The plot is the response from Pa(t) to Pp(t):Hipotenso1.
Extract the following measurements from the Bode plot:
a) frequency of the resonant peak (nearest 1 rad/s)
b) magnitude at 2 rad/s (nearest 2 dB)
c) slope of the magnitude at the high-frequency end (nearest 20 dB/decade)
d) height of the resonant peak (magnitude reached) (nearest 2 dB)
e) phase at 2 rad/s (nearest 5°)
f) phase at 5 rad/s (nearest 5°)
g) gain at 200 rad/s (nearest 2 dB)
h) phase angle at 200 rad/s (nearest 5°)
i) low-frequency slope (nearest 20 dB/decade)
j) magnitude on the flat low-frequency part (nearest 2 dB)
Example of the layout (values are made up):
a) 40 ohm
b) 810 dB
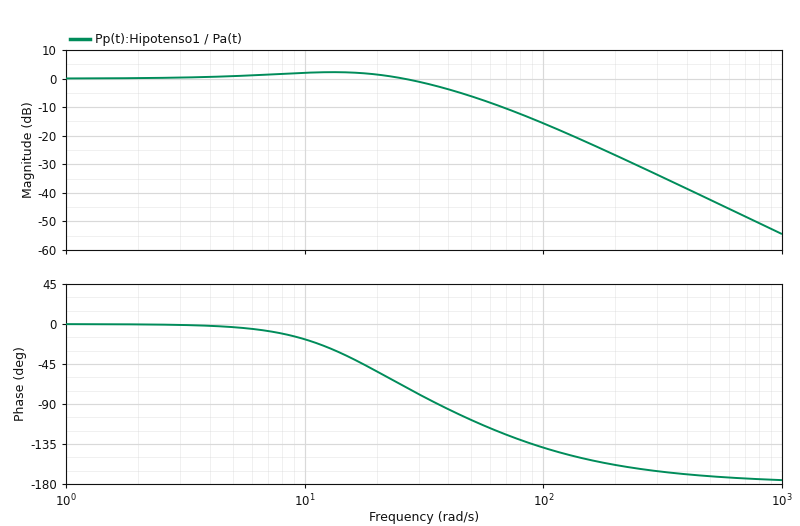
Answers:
a) 13 rad/s
b) 0 dB
c) -40 dB/decade
d) 2 dB
e) 0°
f) -5°
g) -26 dB
h) -160°
i) 0 dB/decade
j) 0 dB
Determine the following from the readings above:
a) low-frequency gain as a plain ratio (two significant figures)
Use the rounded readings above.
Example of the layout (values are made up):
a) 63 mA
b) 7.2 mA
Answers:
a) 1.0
